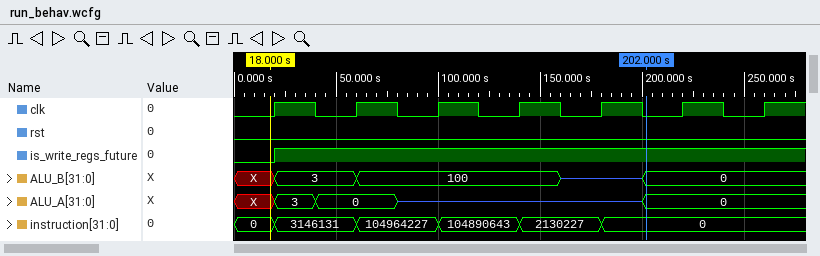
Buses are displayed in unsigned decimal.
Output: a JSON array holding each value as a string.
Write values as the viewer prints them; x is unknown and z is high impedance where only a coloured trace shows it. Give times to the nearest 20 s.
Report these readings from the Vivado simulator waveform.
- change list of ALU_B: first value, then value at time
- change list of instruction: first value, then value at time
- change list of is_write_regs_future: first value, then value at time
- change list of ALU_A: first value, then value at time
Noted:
["X, 3 at 20 s, 100 at 60 s, z at 160 s, 0 at 200 s", "0, 3146131 at 20 s, 104964227 at 60 s, 104890643 at 100 s, 2130227 at 140 s, 0 at 180 s", "0, 1 at 20 s", "X, 3 at 20 s, 0 at 40 s, z at 80 s, 0 at 200 s"]
